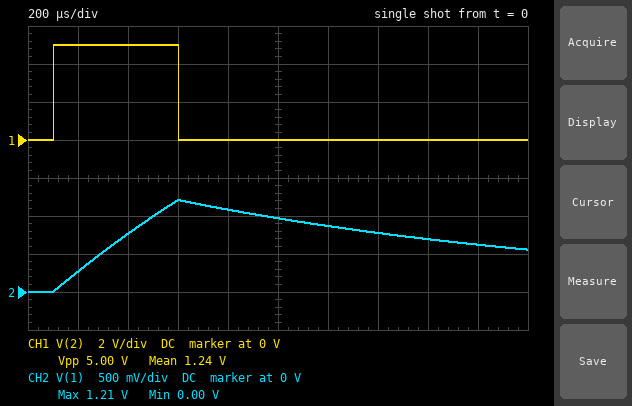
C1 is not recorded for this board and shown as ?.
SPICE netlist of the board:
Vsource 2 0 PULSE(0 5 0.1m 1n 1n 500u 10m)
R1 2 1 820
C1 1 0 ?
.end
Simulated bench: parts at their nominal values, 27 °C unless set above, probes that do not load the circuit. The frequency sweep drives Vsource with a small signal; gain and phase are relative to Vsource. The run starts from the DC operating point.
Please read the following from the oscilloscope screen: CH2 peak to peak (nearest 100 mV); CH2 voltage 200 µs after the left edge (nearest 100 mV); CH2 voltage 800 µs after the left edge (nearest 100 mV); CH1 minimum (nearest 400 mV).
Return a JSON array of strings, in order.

["1.2 V", "300 mV", "1.1 V", "0 V"]
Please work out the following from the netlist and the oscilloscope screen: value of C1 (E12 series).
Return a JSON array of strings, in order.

["2.2 µF"]
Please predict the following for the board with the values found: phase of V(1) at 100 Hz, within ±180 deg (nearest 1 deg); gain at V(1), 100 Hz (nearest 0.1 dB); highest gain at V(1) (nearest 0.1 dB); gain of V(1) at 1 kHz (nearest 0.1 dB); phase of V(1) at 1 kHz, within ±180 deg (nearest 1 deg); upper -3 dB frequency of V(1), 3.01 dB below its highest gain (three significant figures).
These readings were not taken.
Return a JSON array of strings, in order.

["-49 deg", "-3.6 dB", "0 dB", "-21.1 dB", "-85 deg", "88.2 Hz"]
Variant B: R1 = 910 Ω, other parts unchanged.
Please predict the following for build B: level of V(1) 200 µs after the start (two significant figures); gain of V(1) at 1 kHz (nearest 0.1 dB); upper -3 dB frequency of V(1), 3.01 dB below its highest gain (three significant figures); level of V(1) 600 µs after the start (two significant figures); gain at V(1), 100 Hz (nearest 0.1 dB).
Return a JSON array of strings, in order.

["240 mV", "-22.0 dB", "79.5 Hz", "1.1 V", "-4.1 dB"]
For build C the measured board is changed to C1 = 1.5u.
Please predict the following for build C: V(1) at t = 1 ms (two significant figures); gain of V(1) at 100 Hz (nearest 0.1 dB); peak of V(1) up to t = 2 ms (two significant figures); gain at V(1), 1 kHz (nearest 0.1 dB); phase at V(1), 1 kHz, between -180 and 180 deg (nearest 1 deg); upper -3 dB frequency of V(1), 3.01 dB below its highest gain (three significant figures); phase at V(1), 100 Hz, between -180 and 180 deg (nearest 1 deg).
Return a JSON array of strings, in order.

["1.2 V", "-2.0 dB", "1.7 V", "-17.8 dB", "-83 deg", "129 Hz", "-38 deg"]
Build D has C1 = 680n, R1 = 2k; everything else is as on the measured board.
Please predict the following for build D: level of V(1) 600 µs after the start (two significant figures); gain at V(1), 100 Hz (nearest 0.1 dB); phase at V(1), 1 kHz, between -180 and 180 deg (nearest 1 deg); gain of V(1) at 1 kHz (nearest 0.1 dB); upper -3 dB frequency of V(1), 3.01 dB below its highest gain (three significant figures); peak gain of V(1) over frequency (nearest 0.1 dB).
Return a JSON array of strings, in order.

["1.5 V", "-2.4 dB", "-83 deg", "-18.7 dB", "117 Hz", "0 dB"]
